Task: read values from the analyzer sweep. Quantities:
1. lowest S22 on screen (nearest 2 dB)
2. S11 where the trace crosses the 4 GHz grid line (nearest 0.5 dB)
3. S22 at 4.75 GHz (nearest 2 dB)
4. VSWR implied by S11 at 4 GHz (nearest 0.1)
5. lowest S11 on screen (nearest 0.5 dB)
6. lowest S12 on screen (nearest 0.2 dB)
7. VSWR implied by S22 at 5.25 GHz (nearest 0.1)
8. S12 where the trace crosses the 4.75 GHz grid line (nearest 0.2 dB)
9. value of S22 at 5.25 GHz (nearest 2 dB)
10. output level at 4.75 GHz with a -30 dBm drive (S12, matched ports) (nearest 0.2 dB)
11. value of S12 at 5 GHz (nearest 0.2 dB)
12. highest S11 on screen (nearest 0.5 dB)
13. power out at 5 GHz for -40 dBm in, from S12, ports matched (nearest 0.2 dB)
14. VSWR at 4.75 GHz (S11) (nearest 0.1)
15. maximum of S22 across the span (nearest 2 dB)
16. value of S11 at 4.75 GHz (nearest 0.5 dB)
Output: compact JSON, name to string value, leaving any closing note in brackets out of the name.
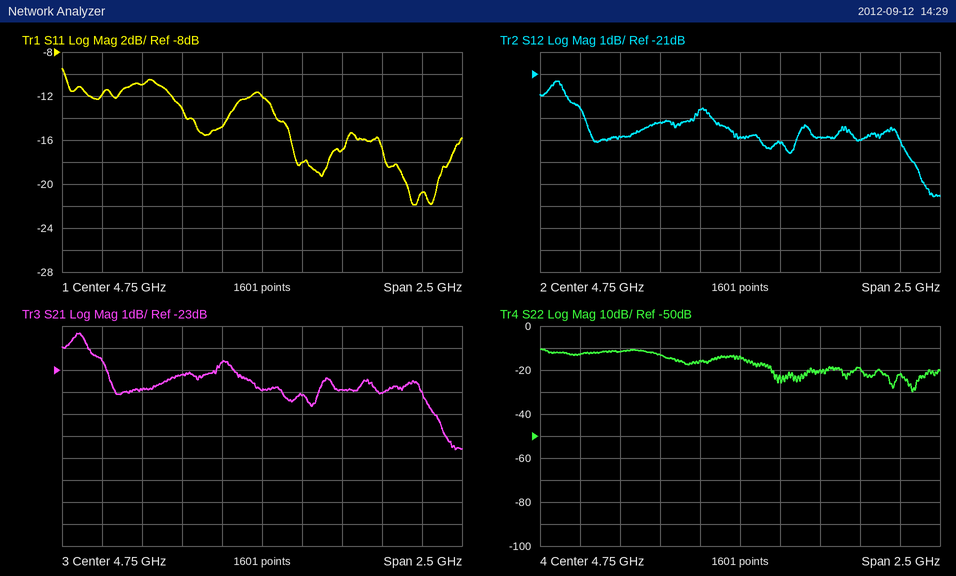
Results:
{"lowest S22 on screen": "-30 dB", "S11 where the trace crosses the 4 GHz grid line": "-11.0 dB", "S22 at 4.75 GHz": "-14 dB", "VSWR implied by S11 at 4 GHz": "1.8", "lowest S11 on screen": "-22.0 dB", "lowest S12 on screen": "-26.6 dB", "VSWR implied by S22 at 5.25 GHz": "1.2", "S12 where the trace crosses the 4.75 GHz grid line": "-23.8 dB", "value of S22 at 5.25 GHz": "-20 dB", "output level at 4.75 GHz with a -30 dBm drive (S12, matched ports)": "-53.8 dBm", "value of S12 at 5 GHz": "-24.2 dB", "highest S11 on screen": "-9.5 dB", "power out at 5 GHz for -40 dBm in, from S12, ports matched": "-64.2 dBm", "VSWR at 4.75 GHz (S11)": "1.7", "maximum of S22 across the span": "-10 dB", "value of S11 at 4.75 GHz": "-12.0 dB"}
